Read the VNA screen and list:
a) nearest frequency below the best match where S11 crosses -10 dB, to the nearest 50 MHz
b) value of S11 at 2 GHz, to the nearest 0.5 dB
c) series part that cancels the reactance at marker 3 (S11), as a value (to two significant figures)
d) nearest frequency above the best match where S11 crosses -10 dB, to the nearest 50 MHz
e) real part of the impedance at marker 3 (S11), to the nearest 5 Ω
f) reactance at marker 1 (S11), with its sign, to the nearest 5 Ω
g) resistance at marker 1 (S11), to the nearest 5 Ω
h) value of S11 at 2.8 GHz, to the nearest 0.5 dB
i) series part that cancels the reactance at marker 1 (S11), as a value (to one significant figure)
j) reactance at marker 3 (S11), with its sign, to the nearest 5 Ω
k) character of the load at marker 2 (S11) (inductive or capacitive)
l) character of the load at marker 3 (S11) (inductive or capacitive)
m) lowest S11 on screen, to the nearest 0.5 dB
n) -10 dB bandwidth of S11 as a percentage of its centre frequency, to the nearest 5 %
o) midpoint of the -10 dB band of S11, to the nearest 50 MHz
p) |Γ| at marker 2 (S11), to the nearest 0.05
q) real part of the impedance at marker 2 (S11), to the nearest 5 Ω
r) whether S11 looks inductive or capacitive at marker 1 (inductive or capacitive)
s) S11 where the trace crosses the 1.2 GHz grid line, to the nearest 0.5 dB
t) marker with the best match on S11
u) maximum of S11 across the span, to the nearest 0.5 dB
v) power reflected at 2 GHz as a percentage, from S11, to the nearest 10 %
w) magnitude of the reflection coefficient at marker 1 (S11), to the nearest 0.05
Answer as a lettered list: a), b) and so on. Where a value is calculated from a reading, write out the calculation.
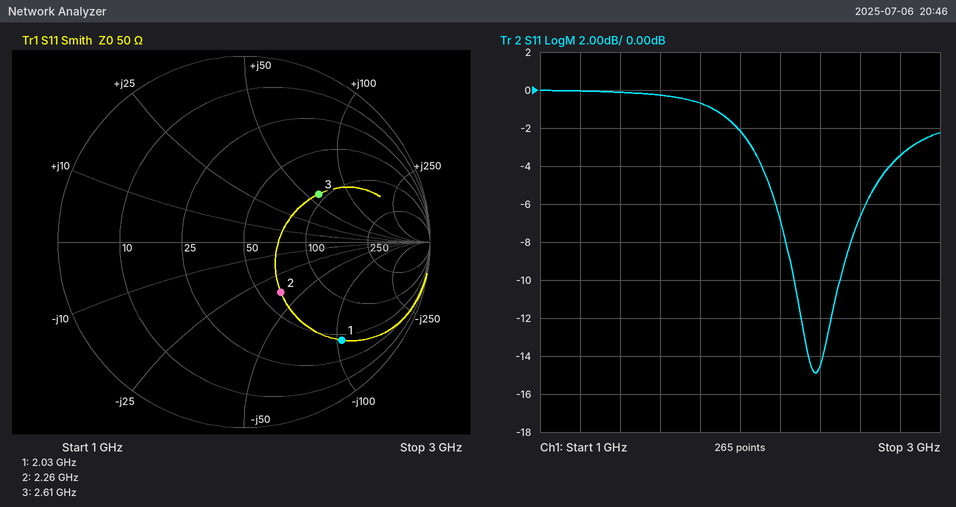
a) 2.25 GHz
b) -2.0 dB
c) C = 1/(2π × 2.61 GHz × 60 Ω) ≈ 1.0 pF
d) 2.50 GHz
e) 90 Ω
f) -105 Ω
g) 45 Ω
h) -3.5 dB
i) L = 105 Ω/(2π × 2.03 GHz) ≈ 8 nH
j) +60 Ω
k) capacitive
l) inductive
m) -15.0 dB
n) 250 MHz / 2.375 GHz ≈ 10 %
o) 2.40 GHz
p) 0.35
q) 60 Ω
r) capacitive
s) 0.0 dB
t) marker 2
u) 0.0 dB
v) 10^(-2/10) ≈ 63.1 %, so 60 % to the nearest 10 %
w) 0.75
